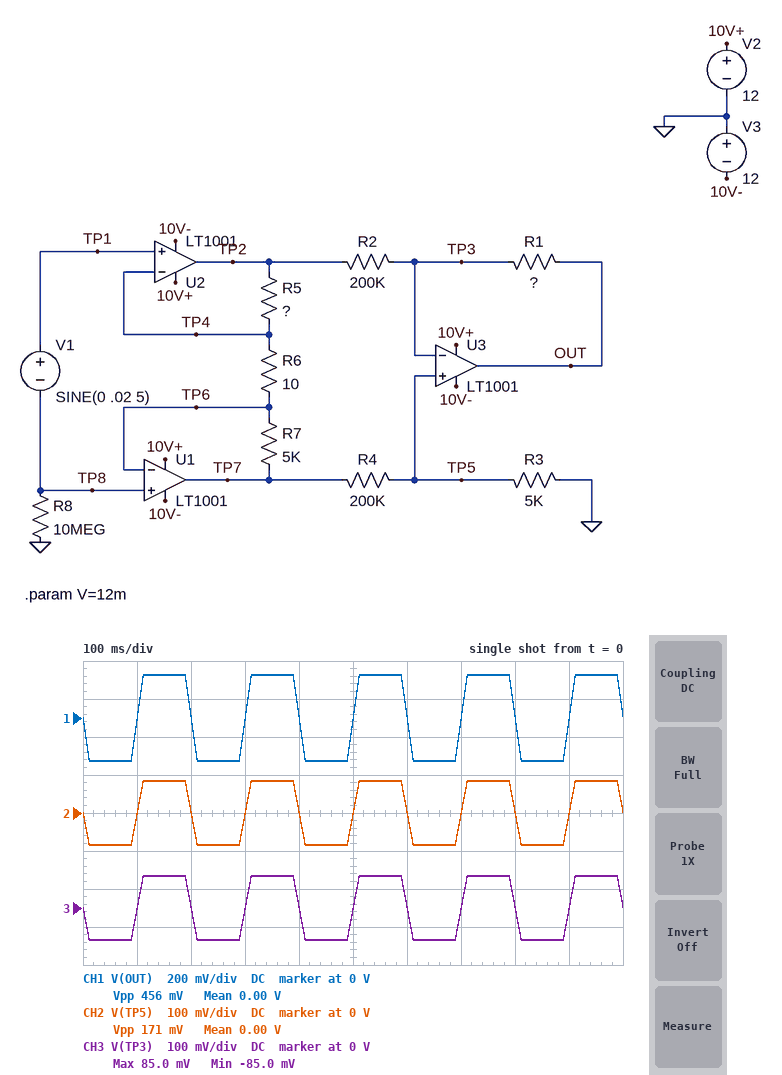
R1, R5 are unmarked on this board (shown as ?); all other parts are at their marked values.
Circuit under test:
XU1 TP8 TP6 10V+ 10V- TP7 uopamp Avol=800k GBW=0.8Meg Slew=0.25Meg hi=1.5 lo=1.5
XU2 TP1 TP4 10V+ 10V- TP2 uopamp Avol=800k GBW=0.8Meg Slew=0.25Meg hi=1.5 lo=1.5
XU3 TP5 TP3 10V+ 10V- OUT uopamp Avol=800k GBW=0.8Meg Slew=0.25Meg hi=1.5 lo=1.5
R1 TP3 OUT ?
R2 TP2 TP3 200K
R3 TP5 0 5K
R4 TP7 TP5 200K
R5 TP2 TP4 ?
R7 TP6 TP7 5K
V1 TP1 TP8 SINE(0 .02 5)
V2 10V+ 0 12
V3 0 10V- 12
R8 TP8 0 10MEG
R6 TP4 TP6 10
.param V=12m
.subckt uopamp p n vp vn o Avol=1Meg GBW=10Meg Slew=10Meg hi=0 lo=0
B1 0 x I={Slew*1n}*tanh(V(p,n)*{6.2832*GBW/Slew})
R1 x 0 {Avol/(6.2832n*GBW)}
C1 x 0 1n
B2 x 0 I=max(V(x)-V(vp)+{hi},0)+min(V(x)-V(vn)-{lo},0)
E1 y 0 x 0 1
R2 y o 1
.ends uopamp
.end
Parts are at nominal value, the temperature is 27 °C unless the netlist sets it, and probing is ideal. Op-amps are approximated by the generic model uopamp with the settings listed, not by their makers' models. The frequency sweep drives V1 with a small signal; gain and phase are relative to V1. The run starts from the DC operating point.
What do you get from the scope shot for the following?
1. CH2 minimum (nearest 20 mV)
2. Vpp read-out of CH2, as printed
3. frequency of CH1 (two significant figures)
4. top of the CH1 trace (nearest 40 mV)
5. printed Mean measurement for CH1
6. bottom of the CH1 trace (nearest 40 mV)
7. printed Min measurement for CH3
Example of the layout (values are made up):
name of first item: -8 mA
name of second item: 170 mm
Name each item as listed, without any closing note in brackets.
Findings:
CH2 minimum: -80 mV
Vpp read-out of CH2, as printed: 171 mV
frequency of CH1: 5.0 Hz
top of the CH1 trace: 240 mV
printed Mean measurement for CH1: 0.00 V
bottom of the CH1 trace: -240 mV
printed Min measurement for CH3: -85.0 mV
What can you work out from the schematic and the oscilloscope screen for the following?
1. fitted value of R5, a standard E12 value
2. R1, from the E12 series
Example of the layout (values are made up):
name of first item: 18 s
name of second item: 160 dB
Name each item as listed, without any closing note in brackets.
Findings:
fitted value of R5, a standard E12 value: 15 kΩ
R1, from the E12 series: 2.7 kΩ
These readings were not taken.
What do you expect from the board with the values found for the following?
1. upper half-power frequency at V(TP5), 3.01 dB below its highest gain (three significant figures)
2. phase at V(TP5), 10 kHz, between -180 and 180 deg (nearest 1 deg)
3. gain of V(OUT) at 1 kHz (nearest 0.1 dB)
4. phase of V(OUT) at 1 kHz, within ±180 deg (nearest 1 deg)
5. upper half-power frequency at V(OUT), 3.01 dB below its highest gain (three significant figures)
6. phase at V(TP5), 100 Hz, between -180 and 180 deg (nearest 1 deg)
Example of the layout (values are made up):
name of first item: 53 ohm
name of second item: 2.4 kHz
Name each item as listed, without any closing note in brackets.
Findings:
upper half-power frequency at V(TP5), 3.01 dB below its highest gain: 401 Hz
phase at V(TP5), 10 kHz, between -180 and 180 deg: 92 deg
gain of V(OUT) at 1 kHz: 21.7 dB
phase of V(OUT) at 1 kHz, within ±180 deg: 112 deg
upper half-power frequency at V(OUT), 3.01 dB below its highest gain: 401 Hz
phase at V(TP5), 100 Hz, between -180 and 180 deg: 166 deg
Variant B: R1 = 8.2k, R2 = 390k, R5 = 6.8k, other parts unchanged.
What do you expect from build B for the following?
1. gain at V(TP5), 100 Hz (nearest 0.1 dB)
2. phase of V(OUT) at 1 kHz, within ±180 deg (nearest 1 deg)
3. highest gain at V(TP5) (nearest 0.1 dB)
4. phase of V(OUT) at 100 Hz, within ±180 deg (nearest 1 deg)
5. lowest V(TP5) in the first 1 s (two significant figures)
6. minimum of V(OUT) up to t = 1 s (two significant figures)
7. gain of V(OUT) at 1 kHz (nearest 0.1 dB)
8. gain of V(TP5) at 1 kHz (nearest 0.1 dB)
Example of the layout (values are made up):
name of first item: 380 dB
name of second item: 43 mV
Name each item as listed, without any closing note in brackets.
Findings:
gain at V(TP5), 100 Hz: 21.6 dB
phase of V(OUT) at 1 kHz, within ±180 deg: 124 deg
highest gain at V(TP5): 21.7 dB
phase of V(OUT) at 100 Hz, within ±180 deg: 172 deg
lowest V(TP5) in the first 1 s: -190 mV
minimum of V(OUT) up to t = 1 s: -410 mV
gain of V(OUT) at 1 kHz: 23.5 dB
gain of V(TP5) at 1 kHz: 16.7 dB
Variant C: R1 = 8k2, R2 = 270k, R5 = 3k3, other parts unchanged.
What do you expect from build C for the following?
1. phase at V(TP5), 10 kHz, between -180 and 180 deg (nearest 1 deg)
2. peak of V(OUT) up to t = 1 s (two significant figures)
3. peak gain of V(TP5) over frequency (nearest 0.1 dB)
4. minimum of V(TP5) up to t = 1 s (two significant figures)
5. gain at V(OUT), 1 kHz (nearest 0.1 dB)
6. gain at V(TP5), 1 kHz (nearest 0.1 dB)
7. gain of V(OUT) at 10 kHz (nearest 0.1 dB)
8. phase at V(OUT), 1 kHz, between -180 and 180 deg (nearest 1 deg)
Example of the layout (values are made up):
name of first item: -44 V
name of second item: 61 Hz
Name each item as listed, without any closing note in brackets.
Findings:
phase at V(TP5), 10 kHz, between -180 and 180 deg: 95 deg
peak of V(OUT) up to t = 1 s: 450 mV
peak gain of V(TP5) over frequency: 21.7 dB
minimum of V(TP5) up to t = 1 s: -240 mV
gain at V(OUT), 1 kHz: 23.9 dB
gain at V(TP5), 1 kHz: 18.5 dB
gain of V(OUT) at 10 kHz: 6.7 dB
phase at V(OUT), 1 kHz, between -180 and 180 deg: 134 deg
